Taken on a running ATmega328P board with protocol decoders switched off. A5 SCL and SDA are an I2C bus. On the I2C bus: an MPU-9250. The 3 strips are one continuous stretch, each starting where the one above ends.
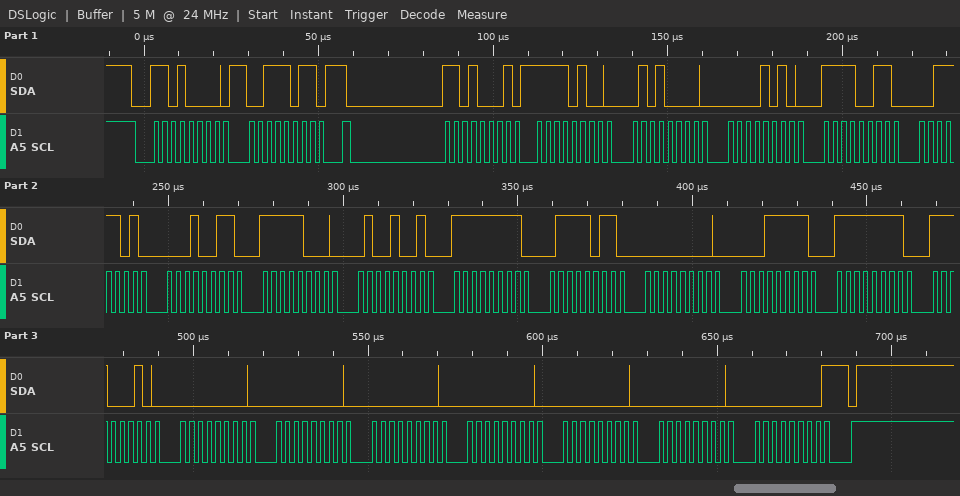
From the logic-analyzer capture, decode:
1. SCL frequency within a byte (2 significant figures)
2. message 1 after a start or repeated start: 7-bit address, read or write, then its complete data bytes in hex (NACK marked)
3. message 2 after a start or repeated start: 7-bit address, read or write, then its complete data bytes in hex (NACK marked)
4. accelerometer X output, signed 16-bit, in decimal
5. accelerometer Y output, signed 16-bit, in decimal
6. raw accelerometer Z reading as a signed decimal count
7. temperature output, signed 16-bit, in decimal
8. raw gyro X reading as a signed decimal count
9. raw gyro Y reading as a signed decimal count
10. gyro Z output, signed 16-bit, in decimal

400 kHz
0x68 write: 3B
0x68 read: F4 50 0A F3 3D 13 F8 49 FF 7B 00 1F FF E2 00 00 00 00 00 00 00 NACK
-2992
2803
15635
-1975
-133
31
-30
